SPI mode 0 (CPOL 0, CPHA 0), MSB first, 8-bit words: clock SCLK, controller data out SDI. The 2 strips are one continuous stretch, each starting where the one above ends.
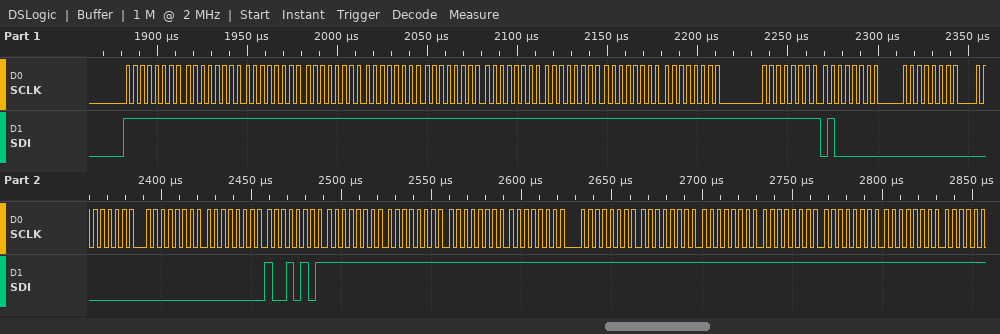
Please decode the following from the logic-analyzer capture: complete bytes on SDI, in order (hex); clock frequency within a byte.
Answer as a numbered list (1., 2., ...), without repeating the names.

1. FF FF FF FF FF FF FF FF FF FF FF 40 00 00 00 00 95 FF FF FF FF FF FF FF FF FF FF
2. 250 kHz
